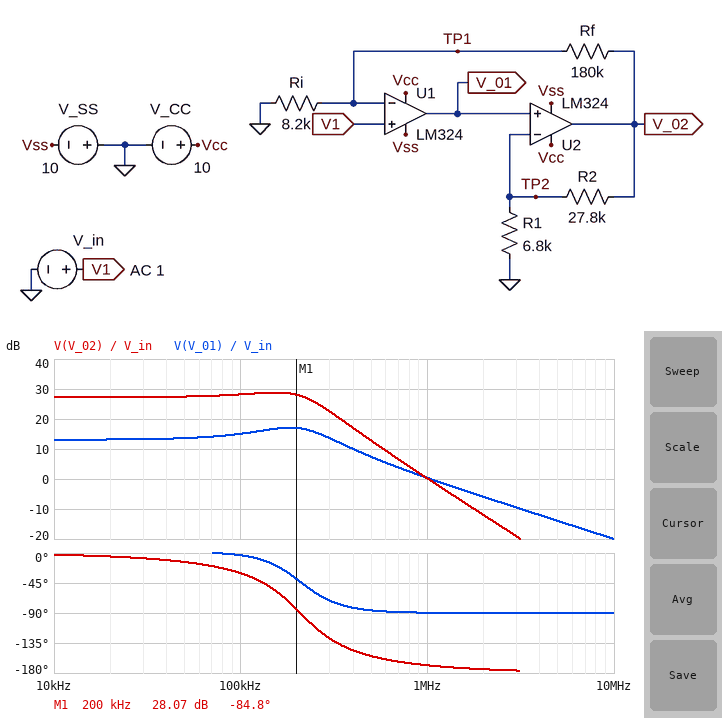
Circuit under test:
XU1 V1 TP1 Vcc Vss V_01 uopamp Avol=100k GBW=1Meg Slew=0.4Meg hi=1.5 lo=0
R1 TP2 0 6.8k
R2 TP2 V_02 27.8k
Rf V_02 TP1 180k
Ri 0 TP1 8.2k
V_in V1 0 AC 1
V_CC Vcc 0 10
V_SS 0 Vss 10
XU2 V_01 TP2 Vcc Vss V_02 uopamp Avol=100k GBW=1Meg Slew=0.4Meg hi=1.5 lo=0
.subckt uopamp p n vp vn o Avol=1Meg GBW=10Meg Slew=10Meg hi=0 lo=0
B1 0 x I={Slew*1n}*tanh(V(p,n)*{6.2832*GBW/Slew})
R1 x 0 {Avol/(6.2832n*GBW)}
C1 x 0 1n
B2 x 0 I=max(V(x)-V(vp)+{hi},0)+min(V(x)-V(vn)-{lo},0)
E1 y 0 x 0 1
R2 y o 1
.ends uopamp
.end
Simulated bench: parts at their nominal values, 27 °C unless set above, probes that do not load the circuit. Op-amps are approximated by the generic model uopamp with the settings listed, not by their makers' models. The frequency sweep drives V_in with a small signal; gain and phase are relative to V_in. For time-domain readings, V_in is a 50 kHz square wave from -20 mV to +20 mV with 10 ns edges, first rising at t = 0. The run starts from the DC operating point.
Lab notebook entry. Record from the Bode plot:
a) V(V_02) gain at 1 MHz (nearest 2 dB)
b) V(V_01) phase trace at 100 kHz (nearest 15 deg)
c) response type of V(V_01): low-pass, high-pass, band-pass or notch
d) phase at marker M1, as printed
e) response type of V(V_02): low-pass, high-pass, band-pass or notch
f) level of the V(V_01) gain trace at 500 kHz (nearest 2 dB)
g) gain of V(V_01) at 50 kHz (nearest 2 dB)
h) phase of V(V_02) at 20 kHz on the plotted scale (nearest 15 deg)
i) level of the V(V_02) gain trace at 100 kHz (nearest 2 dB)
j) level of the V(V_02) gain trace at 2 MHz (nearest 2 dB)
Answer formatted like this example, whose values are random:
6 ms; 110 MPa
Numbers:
0 dB; 0 deg; low-pass; -84.8 deg; low-pass; 8 dB; 14 dB; 0 deg; 28 dB; -12 dB
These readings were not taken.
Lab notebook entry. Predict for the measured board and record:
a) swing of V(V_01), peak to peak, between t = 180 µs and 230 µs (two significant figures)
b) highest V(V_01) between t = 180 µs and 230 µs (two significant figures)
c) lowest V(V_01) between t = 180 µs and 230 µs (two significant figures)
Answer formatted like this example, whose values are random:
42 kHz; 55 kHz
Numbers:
480 mV; 240 mV; -240 mV
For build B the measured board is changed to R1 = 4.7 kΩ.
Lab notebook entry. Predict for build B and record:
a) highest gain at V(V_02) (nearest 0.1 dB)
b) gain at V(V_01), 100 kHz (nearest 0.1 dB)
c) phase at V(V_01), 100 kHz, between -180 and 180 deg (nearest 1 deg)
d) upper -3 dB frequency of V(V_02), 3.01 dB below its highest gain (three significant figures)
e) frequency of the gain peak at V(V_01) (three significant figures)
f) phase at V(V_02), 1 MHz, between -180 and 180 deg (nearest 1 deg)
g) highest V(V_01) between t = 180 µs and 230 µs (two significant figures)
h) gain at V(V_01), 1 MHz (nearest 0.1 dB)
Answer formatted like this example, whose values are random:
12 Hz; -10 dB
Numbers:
31.0 dB; 13.6 dB; 11 deg; 248 kHz; 200 kHz; -171 deg; 290 mV; 0.4 dB
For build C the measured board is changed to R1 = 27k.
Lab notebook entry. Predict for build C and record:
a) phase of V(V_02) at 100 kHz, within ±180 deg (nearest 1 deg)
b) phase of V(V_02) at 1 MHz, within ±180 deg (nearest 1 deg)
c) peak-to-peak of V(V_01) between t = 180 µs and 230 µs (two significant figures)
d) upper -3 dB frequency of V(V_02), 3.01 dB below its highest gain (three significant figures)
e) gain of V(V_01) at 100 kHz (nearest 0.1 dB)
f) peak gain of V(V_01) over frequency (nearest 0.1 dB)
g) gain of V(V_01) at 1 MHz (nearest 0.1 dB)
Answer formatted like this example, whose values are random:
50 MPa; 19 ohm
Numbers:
-56 deg; -153 deg; 450 mV; 107 kHz; 18.5 dB; 21.1 dB; 0.3 dB
